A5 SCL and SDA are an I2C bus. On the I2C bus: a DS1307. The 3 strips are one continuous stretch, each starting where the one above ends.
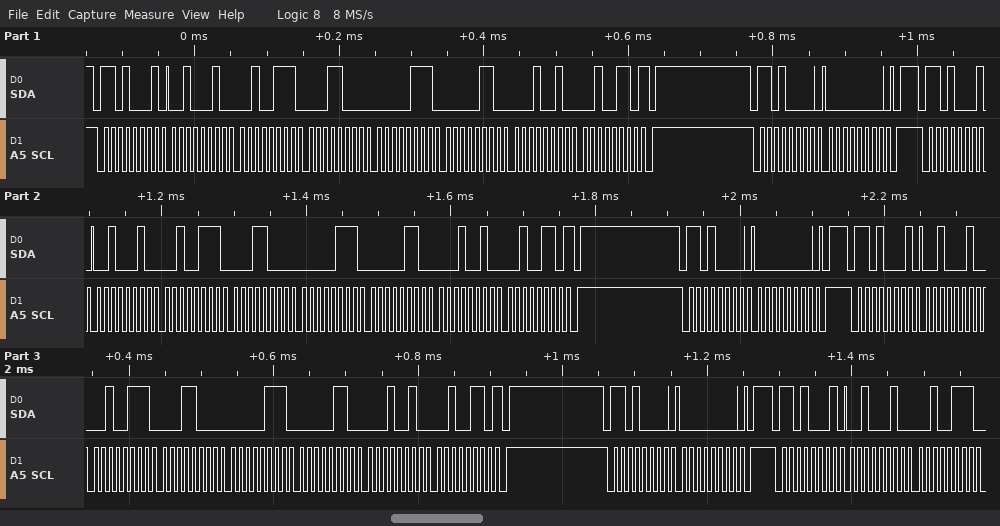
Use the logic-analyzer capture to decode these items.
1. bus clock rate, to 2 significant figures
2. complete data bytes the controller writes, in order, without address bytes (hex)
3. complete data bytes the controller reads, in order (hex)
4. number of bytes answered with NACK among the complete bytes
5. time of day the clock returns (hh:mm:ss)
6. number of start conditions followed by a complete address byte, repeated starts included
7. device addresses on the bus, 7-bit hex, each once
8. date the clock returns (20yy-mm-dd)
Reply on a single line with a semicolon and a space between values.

100 kHz; 00 00 00; 22 27 18 07 06 12 26 22 27 18 07 06 12 26 22 27 18 07 06 12 26 22 27; 3; 18:27:22; 7; 0x68; 2026-12-06
